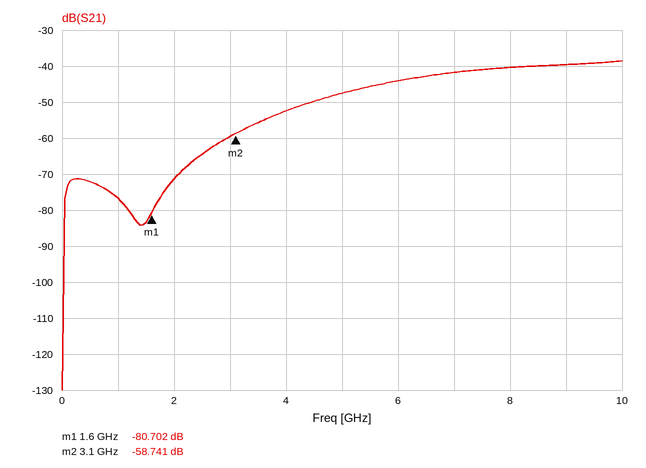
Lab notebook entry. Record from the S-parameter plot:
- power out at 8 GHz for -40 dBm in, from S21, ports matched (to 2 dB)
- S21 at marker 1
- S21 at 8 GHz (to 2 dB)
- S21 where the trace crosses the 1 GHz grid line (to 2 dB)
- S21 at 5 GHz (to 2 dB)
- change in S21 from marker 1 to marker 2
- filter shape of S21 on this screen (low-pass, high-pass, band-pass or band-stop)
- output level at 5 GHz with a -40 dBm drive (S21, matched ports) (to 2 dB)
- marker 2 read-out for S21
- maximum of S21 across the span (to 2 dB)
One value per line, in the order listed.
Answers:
-80 dBm
-80.702 dB
-40 dB
-76 dB
-48 dB
21.961 dB
high-pass
-88 dBm
-58.741 dB
-38 dB
